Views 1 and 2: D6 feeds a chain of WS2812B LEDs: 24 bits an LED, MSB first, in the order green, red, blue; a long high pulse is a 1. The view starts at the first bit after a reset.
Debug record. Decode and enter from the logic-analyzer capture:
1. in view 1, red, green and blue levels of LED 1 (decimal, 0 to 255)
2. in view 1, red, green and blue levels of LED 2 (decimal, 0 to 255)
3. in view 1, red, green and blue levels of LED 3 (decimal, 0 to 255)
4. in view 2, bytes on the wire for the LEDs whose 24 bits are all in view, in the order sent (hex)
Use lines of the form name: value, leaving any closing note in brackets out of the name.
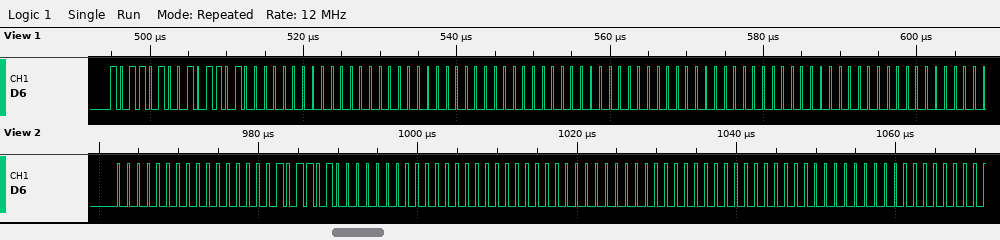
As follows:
in view 1, red, green and blue levels of LED 1: 180, 180, 0
in view 1, red, green and blue levels of LED 2: 0, 0, 0
in view 1, red, green and blue levels of LED 3: 0, 0, 0
in view 2, bytes on the wire for the LEDs whose 24 bits are all in view, in the order sent: 00 00 B4 00 00 00 00 00 00
